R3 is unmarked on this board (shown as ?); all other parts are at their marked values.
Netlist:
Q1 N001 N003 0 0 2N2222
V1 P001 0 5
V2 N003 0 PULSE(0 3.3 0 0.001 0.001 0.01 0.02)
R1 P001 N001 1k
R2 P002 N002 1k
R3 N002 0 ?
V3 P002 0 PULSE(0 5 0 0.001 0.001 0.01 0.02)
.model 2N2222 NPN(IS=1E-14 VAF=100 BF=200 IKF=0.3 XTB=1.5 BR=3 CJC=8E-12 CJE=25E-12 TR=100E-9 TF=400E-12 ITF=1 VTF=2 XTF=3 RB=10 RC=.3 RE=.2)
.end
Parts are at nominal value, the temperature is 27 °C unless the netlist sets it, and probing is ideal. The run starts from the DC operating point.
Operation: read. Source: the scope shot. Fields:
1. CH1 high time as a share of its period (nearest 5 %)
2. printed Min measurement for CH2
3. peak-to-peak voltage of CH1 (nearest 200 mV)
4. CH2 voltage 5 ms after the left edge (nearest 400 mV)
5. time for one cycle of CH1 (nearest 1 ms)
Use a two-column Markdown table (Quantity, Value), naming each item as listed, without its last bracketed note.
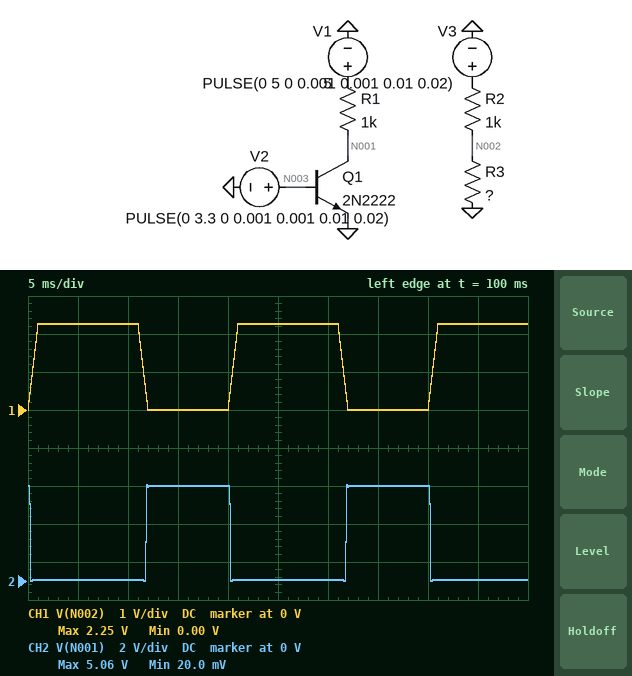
| Quantity | Value |
|---|---|
| CH1 high time as a share of its period | 55 % |
| printed Min measurement for CH2 | 20.0 mV |
| peak-to-peak voltage of CH1 | 2.2 V |
| CH2 voltage 5 ms after the left edge | 0 V |
| time for one cycle of CH1 | 20 ms |
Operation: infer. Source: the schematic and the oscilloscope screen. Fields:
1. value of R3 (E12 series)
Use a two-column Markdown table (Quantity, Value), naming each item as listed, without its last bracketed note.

| Quantity | Value |
|---|---|
| value of R3 | 820 Ω |
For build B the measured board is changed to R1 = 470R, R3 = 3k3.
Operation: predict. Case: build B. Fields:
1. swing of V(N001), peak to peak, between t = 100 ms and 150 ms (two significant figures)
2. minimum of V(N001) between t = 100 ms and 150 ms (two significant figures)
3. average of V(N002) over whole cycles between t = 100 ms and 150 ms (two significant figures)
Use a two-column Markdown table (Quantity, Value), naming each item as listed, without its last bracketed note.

| Quantity | Value |
|---|---|
| swing of V(N001), peak to peak, between t = 100 ms and 150 ms | 5.0 V |
| minimum of V(N001) between t = 100 ms and 150 ms | 22 mV |
| average of V(N002) over whole cycles between t = 100 ms and 150 ms | 2.1 V |
